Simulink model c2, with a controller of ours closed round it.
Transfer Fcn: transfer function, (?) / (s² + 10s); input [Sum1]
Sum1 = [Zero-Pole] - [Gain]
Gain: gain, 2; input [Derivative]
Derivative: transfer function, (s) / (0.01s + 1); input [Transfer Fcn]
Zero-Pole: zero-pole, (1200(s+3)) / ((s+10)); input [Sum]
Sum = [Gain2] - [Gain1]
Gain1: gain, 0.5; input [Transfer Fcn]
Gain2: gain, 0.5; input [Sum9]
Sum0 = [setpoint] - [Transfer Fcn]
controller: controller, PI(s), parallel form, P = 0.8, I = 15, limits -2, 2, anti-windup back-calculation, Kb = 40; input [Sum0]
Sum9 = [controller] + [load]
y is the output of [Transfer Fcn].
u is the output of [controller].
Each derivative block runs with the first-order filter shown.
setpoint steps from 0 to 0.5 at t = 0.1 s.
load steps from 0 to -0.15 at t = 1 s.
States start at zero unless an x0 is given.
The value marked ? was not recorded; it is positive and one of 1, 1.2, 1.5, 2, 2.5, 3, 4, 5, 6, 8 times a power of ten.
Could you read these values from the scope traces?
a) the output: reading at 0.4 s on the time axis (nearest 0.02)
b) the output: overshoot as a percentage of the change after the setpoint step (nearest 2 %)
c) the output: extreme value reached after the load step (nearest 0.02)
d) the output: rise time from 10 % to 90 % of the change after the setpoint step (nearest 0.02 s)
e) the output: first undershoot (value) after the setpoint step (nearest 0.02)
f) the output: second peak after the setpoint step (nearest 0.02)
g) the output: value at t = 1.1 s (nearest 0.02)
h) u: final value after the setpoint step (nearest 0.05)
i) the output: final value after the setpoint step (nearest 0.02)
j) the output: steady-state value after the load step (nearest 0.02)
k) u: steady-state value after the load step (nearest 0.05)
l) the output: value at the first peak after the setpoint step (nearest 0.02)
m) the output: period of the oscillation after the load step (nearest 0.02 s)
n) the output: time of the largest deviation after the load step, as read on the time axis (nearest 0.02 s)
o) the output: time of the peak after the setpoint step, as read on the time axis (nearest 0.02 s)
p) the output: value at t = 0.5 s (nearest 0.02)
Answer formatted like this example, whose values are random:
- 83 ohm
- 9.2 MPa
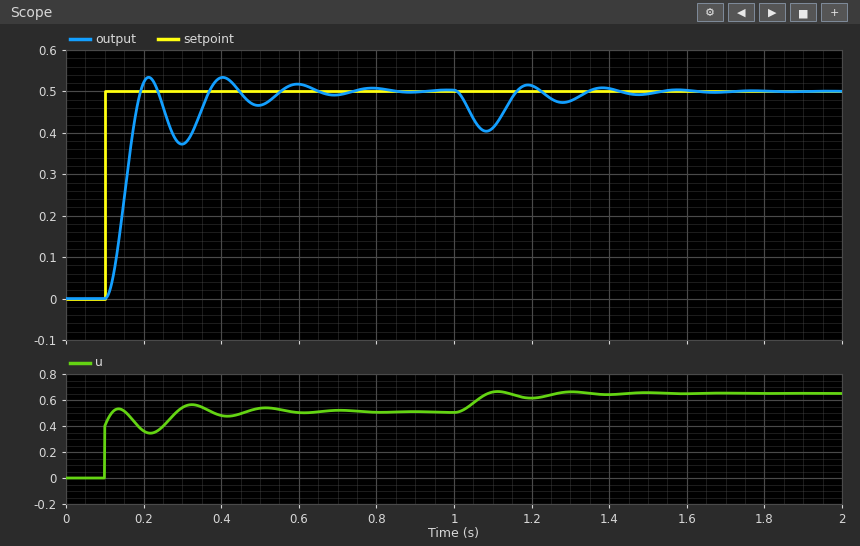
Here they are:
- 0.54
- 6 %
- 0.40
- 0.06 s
- 0.38
- 0.54
- 0.42
- 0.50
- 0.50
- 0.50
- 0.65
- 0.54
- 0.20 s
- 1.08 s
- 0.22 s
- 0.46
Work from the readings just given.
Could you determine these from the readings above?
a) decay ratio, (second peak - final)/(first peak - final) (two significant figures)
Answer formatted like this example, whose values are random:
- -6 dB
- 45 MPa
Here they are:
- 1.0
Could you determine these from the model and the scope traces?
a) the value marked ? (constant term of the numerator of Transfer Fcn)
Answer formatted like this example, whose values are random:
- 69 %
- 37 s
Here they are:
- 1
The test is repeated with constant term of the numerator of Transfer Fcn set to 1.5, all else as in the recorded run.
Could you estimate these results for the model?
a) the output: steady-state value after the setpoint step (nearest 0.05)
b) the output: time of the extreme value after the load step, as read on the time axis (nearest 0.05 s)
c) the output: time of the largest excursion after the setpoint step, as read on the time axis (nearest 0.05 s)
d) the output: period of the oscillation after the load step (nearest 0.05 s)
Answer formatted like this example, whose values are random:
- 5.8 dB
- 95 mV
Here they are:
- 0.50
- 1.05 s
- 0.35 s
- 0.15 s
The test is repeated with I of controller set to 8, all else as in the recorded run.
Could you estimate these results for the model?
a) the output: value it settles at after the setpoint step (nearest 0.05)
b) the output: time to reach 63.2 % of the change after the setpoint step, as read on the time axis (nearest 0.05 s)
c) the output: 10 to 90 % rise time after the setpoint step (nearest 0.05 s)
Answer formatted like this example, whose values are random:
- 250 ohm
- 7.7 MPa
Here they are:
- 0.50
- 0.15 s
- 0.25 s
